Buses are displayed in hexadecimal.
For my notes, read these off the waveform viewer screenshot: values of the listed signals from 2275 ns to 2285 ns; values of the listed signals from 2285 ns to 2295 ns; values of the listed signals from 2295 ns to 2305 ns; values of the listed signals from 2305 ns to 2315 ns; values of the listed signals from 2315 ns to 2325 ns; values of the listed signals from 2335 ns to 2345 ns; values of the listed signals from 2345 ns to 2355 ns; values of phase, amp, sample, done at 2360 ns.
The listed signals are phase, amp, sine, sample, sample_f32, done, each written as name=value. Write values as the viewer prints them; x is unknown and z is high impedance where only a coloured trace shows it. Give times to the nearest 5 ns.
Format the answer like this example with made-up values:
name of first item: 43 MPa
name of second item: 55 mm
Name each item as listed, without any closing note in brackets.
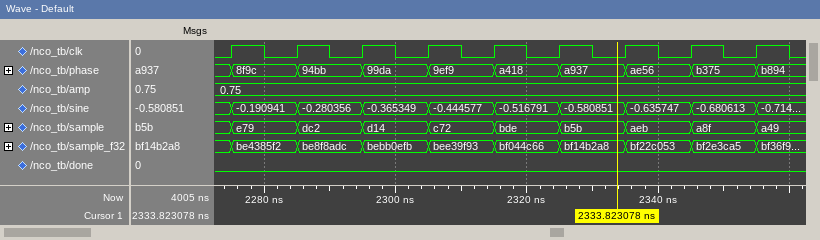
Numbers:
values of the listed signals from 2275 ns to 2285 ns: phase=8f9c, amp=0.75, sine=-0.190941, sample=e79, sample_f32=be4385f2, done=0
values of the listed signals from 2285 ns to 2295 ns: phase=94bb, amp=0.75, sine=-0.280356, sample=dc2, sample_f32=be8f8adc, done=0
values of the listed signals from 2295 ns to 2305 ns: phase=99da, amp=0.75, sine=-0.365349, sample=d14, sample_f32=bebb0efb, done=0
values of the listed signals from 2305 ns to 2315 ns: phase=9ef9, amp=0.75, sine=-0.444577, sample=c72, sample_f32=bee39f93, done=0
values of the listed signals from 2315 ns to 2325 ns: phase=a418, amp=0.75, sine=-0.516791, sample=bde, sample_f32=bf044c66, done=0
values of the listed signals from 2335 ns to 2345 ns: phase=ae56, amp=0.75, sine=-0.635747, sample=aeb, sample_f32=bf22c053, done=0
values of the listed signals from 2345 ns to 2355 ns: phase=b375, amp=0.75, sine=-0.680613, sample=a8f, sample_f32=bf2e3ca5, done=0
values of phase, amp, sample, done at 2360 ns: phase=b894, amp=0.75, sample=a49, done=0
